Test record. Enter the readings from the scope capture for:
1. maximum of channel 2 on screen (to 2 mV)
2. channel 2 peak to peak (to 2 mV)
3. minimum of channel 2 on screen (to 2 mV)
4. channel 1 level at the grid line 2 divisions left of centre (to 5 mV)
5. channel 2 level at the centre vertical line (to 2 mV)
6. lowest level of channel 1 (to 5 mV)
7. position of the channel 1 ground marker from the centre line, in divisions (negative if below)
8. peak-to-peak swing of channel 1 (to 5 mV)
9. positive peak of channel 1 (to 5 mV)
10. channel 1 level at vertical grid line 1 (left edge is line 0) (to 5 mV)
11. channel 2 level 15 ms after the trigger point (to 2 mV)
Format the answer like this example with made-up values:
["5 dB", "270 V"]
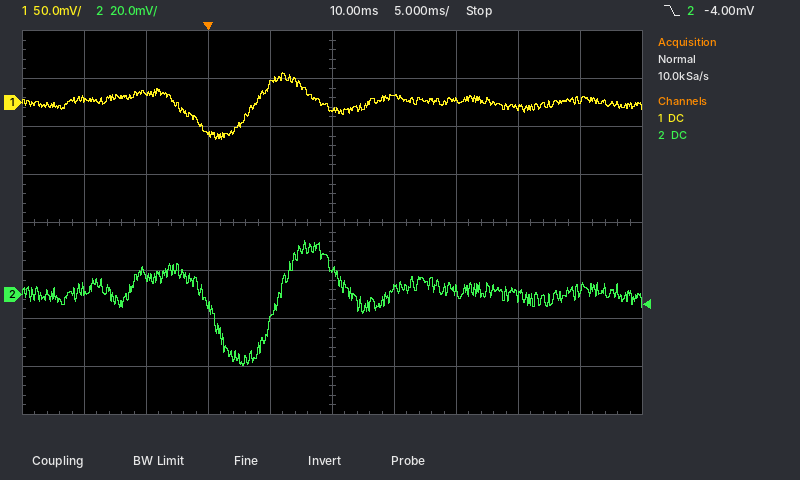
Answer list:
["22 mV", "52 mV", "-30 mV", "-35 mV", "10 mV", "-40 mV", "+2.5 div", "70 mV", "30 mV", "5 mV", "2 mV"]
